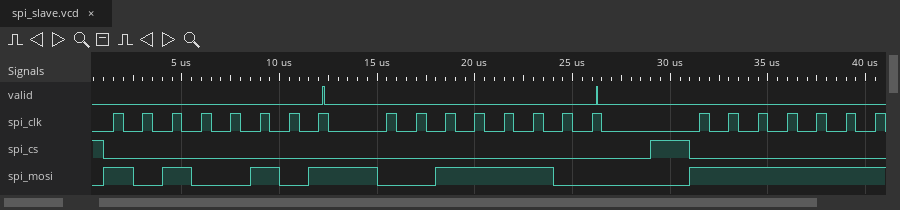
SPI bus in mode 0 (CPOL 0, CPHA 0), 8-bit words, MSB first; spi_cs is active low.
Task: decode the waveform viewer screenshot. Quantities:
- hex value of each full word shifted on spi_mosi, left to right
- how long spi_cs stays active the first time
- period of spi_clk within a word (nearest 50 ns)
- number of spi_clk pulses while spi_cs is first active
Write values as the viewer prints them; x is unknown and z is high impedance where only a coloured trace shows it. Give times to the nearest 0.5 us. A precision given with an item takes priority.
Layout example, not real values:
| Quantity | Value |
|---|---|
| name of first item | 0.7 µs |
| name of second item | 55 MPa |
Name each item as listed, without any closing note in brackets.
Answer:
| Quantity | Value |
|---|---|
| hex value of each full word shifted on spi_mosi, left to right | A5, 3C |
| how long spi_cs stays active the first time | 28 us |
| period of spi_clk within a word | 1500 ns |
| number of spi_clk pulses while spi_cs is first active | 16 |
